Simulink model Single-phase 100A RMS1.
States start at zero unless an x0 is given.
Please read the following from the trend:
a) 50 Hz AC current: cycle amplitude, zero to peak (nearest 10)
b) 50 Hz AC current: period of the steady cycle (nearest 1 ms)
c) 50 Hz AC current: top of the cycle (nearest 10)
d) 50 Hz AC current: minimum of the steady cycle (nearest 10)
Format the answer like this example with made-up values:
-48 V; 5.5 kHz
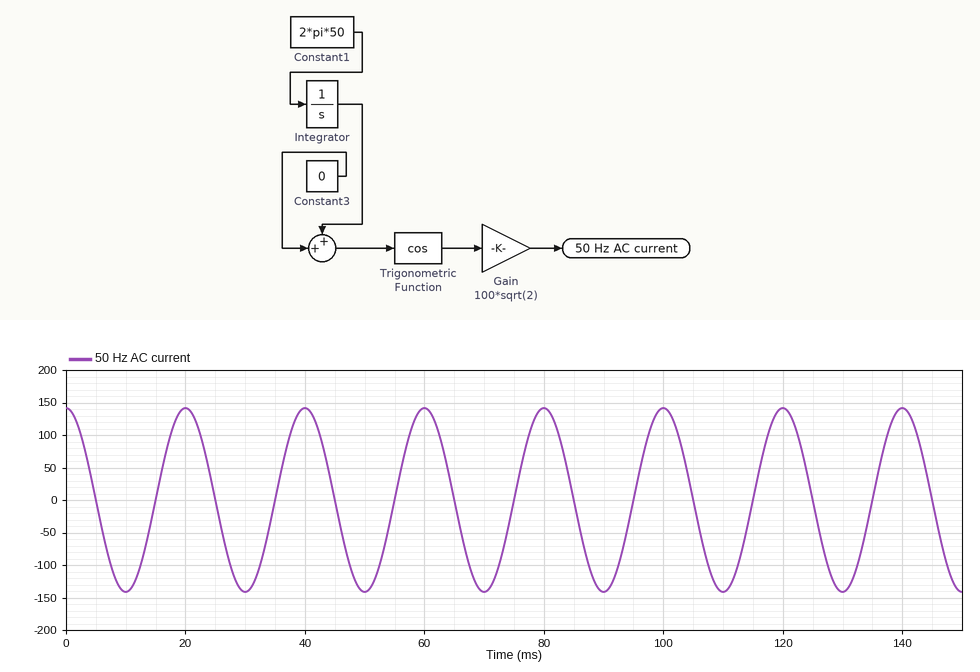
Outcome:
140; 20 ms; 140; -140
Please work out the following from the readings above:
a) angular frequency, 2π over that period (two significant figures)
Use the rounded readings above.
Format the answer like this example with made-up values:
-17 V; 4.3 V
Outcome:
0.31 rad/ms
